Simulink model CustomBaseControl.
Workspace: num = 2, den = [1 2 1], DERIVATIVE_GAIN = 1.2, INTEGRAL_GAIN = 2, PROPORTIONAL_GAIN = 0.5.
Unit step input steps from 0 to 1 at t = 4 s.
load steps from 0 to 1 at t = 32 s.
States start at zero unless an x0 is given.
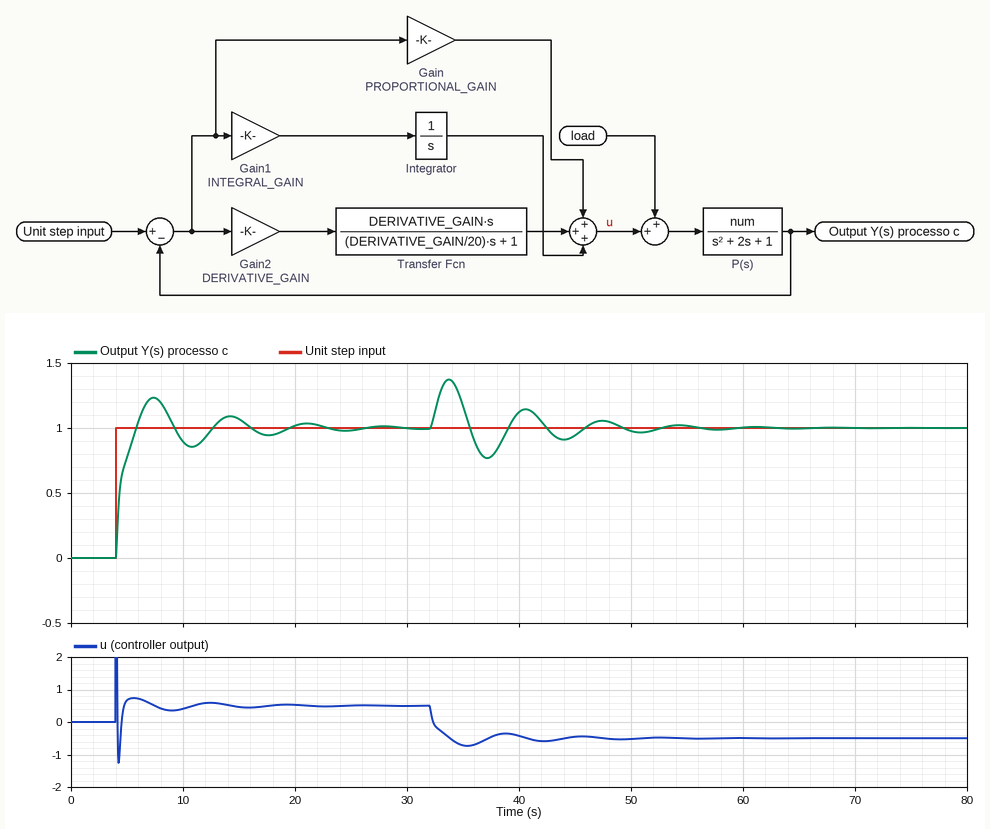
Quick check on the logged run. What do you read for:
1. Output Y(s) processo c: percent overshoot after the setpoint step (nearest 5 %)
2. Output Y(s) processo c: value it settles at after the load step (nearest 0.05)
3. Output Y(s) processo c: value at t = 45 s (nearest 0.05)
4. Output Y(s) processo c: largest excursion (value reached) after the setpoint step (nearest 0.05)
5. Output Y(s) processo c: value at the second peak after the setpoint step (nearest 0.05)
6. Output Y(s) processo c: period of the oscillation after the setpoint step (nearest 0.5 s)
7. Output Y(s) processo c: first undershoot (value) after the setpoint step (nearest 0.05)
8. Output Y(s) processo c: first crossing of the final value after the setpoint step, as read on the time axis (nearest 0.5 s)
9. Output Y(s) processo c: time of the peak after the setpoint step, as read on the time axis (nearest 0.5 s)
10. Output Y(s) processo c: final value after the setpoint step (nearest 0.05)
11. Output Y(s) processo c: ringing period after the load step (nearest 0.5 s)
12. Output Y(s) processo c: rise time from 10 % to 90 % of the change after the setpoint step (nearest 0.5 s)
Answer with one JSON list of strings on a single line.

["25 %", "1.00", "0.95", "1.25", "1.10", "7.0 s", "0.85", "6.0 s", "7.5 s", "1.00", "7.0 s", "1.5 s"]
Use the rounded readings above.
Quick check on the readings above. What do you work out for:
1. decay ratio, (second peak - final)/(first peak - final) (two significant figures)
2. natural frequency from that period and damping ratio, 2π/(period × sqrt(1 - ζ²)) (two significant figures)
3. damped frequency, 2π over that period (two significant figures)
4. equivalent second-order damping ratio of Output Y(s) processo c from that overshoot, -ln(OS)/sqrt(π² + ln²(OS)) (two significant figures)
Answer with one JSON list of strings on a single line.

["0.40", "0.98 rad/s", "0.90 rad/s", "0.40"]
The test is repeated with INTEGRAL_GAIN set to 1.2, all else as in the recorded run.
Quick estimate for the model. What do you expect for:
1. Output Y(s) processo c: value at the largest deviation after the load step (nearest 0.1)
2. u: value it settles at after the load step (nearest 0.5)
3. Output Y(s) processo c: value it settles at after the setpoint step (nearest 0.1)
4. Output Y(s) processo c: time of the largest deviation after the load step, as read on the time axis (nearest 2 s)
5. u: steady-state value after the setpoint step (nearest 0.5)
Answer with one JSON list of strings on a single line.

["1.4", "-0.5", "1.0", "34 s", "0.5"]
